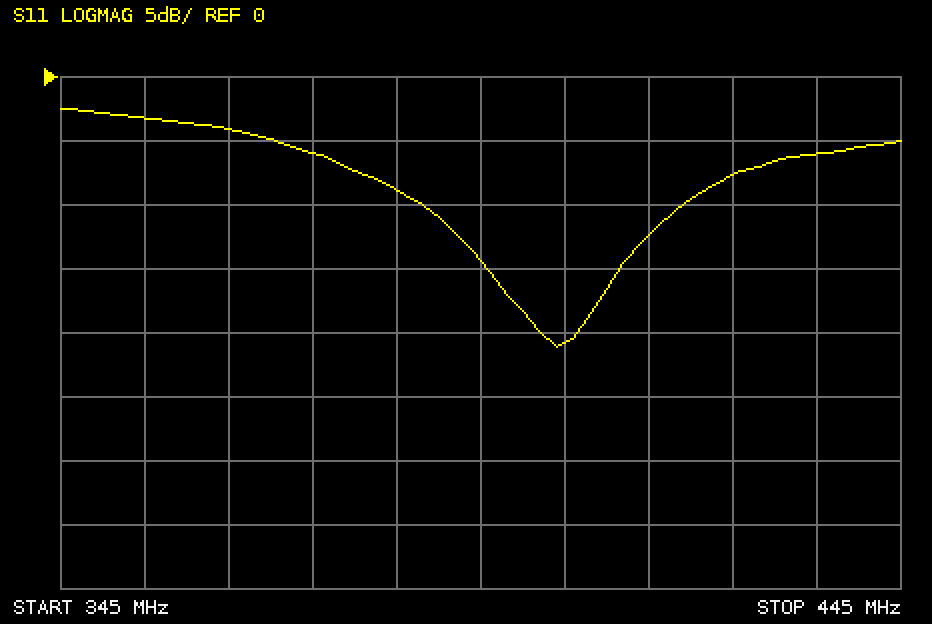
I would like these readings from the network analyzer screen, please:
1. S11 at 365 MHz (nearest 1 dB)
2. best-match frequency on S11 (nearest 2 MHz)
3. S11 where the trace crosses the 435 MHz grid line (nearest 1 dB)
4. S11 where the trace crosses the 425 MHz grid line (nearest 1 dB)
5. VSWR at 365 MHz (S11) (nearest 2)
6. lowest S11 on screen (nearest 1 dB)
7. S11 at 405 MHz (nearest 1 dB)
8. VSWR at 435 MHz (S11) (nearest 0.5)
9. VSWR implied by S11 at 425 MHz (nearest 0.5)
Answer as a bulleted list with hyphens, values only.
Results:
- -4 dB
- 404 MHz
- -6 dB
- -8 dB
- 4
- -21 dB
- -21 dB
- 3.0
- 2.5
